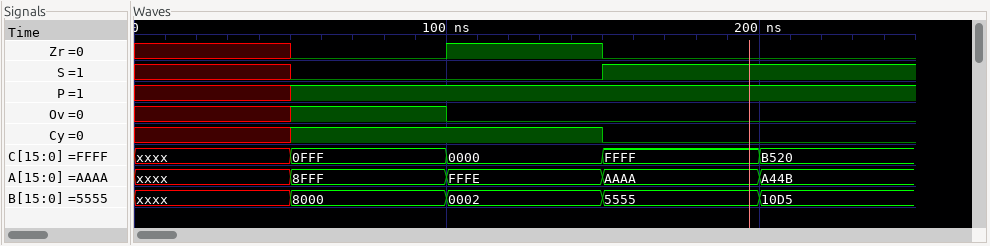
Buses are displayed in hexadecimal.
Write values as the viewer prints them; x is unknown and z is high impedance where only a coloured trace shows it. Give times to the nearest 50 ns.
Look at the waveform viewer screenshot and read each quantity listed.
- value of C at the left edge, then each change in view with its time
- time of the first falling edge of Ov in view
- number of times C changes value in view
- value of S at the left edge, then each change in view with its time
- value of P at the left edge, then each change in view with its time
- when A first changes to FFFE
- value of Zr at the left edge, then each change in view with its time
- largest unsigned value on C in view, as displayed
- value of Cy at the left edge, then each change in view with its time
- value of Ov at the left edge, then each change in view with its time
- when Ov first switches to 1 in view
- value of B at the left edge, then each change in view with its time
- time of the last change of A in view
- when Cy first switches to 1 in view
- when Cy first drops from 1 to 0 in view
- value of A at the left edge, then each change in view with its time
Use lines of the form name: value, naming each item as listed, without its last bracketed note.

value of C at the left edge, then each change in view with its time: xxxx, 0FFF at 50 ns, 0000 at 100 ns, FFFF at 150 ns, B520 at 200 ns
time of the first falling edge of Ov in view: 100 ns
number of times C changes value in view: 4
value of S at the left edge, then each change in view with its time: x, 0 at 50 ns, 1 at 150 ns
value of P at the left edge, then each change in view with its time: x, 1 at 50 ns
when A first changes to FFFE: 100 ns
value of Zr at the left edge, then each change in view with its time: x, 0 at 50 ns, 1 at 100 ns, 0 at 150 ns
largest unsigned value on C in view, as displayed: FFFF
value of Cy at the left edge, then each change in view with its time: x, 1 at 50 ns, 0 at 150 ns
value of Ov at the left edge, then each change in view with its time: x, 1 at 50 ns, 0 at 100 ns
when Ov first switches to 1 in view: 50 ns
value of B at the left edge, then each change in view with its time: xxxx, 8000 at 50 ns, 0002 at 100 ns, 5555 at 150 ns, 10D5 at 200 ns
time of the last change of A in view: 200 ns
when Cy first switches to 1 in view: 50 ns
when Cy first drops from 1 to 0 in view: 150 ns
value of A at the left edge, then each change in view with its time: xxxx, 8FFF at 50 ns, FFFE at 100 ns, AAAA at 150 ns, A44B at 200 ns
